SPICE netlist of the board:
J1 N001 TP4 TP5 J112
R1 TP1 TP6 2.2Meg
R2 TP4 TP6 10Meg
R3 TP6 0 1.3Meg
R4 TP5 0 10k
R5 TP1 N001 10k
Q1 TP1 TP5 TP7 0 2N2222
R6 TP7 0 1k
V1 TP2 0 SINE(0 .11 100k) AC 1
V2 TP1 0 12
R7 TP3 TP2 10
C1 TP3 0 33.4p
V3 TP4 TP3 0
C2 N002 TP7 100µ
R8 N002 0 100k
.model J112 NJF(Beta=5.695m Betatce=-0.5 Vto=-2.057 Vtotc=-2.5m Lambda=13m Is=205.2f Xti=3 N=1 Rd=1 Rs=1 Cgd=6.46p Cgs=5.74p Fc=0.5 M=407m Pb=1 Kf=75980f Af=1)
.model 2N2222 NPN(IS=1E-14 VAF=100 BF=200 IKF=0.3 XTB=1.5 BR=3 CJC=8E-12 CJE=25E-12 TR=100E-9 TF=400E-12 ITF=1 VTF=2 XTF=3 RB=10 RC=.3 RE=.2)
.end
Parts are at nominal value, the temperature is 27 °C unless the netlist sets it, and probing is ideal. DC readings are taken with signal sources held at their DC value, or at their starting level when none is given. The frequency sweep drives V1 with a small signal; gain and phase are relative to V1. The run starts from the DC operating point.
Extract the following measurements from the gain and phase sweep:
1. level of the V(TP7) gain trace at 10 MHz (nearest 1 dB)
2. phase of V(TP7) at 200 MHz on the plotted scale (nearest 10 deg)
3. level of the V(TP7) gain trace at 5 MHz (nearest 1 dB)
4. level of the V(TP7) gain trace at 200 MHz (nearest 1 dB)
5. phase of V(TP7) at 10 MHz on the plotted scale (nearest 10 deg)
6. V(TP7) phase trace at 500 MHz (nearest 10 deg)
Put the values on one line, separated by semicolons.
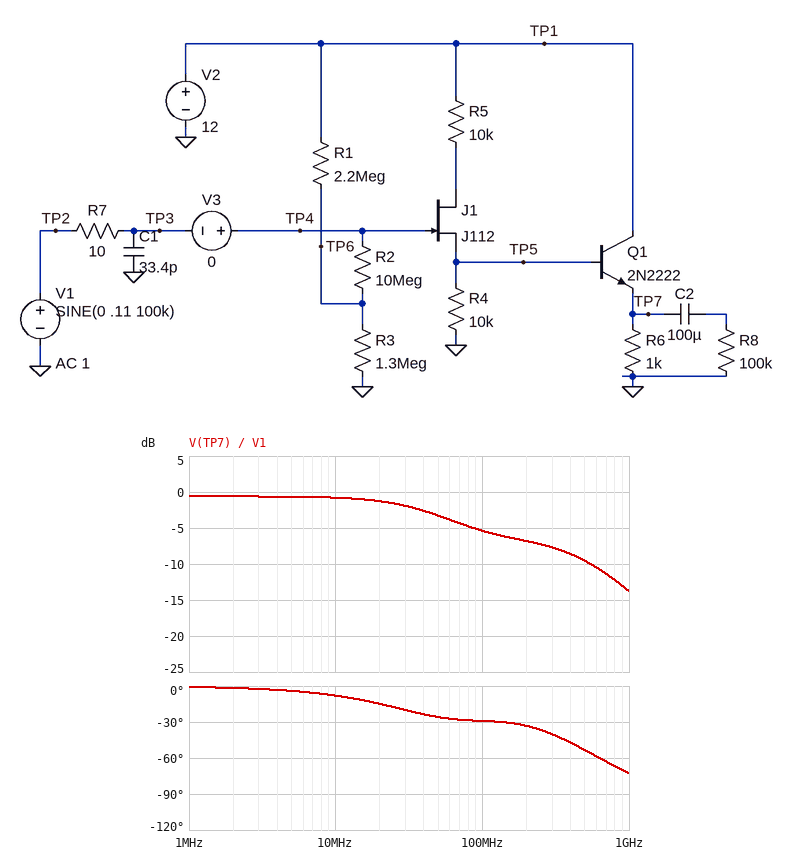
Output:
-1 dB; -30 deg; -1 dB; -7 dB; -10 deg; -50 deg
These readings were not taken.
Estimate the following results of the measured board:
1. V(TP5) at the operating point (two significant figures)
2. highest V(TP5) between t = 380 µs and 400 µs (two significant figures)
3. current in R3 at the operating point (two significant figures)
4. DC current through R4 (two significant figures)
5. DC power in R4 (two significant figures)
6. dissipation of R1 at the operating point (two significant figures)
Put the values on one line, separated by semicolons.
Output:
1.9 V; 2.0 V; 3.2 µA; 190 µA; 350 µW; 28 µW
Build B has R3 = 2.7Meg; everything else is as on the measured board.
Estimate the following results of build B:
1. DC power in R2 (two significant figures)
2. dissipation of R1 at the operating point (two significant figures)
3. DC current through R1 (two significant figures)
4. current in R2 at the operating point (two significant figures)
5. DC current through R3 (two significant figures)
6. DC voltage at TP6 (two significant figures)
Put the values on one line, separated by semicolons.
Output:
3.5 µW; 17 µW; 2.8 µA; 590 nA; 2.2 µA; 5.9 V
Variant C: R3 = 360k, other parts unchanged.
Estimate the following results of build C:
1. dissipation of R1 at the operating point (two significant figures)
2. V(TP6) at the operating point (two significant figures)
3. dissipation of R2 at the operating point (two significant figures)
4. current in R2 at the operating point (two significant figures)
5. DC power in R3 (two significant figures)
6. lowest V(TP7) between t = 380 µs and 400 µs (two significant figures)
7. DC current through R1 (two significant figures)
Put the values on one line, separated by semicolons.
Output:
49 µW; 1.6 V; 270 nW; 160 nA; 7.4 µW; 1.1 V; 4.7 µA
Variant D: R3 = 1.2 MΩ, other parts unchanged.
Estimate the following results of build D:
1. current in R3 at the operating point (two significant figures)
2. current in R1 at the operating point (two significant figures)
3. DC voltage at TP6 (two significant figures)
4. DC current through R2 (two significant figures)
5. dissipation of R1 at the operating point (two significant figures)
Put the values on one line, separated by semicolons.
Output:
3.3 µA; 3.7 µA; 3.9 V; 390 nA; 30 µW
